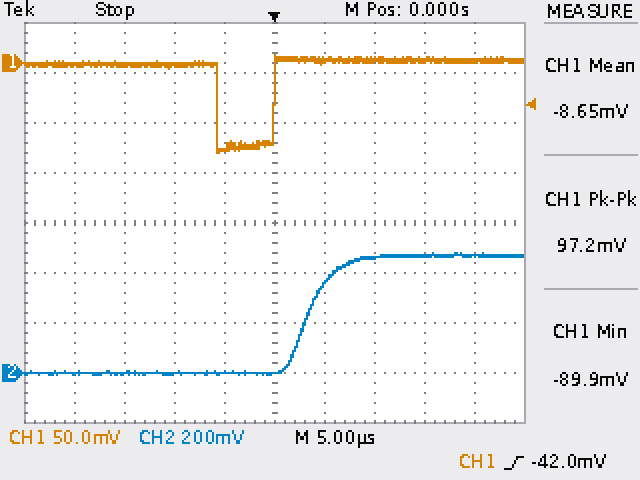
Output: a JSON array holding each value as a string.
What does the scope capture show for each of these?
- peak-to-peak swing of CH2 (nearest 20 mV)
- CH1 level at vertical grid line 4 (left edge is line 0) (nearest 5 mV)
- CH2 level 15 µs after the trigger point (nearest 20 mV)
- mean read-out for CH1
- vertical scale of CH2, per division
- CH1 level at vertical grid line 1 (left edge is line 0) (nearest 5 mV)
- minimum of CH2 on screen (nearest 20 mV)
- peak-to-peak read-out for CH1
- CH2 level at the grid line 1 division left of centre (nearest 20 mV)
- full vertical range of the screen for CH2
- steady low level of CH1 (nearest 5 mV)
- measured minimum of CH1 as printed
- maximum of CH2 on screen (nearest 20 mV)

["480 mV", "-85 mV", "460 mV", "-8.65 mV", "200 mV", "0 mV", "0 mV", "97.2 mV", "0 mV", "1.6 V", "-85 mV", "-89.9 mV", "480 mV"]
